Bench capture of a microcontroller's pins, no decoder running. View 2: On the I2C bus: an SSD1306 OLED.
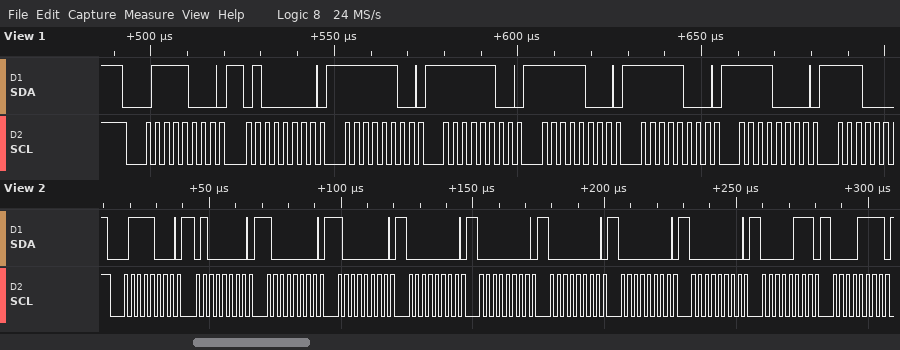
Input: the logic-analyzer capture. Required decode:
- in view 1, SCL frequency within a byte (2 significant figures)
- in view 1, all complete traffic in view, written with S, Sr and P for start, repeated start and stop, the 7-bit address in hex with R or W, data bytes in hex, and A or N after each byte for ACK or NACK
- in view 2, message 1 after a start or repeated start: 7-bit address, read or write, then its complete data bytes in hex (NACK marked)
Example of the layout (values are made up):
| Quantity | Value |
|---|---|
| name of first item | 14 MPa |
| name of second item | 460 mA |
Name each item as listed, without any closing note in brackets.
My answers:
| Quantity | Value |
|---|---|
| in view 1, SCL frequency within a byte | 400 kHz |
| in view 1, all complete traffic in view, written with S, Sr and P for start, repeated start and stop, the 7-bit address in hex with R or W, data bytes in hex, and A or N after each byte for ACK or NACK | S 3CW A 40 A FC A FC A F8 A F8 A F0 A |
| in view 2, message 1 after a start or repeated start: 7-bit address, read or write, then its complete data bytes in hex | 0x3C write: 40 80 80 00 00 00 00 00 07 0F |
